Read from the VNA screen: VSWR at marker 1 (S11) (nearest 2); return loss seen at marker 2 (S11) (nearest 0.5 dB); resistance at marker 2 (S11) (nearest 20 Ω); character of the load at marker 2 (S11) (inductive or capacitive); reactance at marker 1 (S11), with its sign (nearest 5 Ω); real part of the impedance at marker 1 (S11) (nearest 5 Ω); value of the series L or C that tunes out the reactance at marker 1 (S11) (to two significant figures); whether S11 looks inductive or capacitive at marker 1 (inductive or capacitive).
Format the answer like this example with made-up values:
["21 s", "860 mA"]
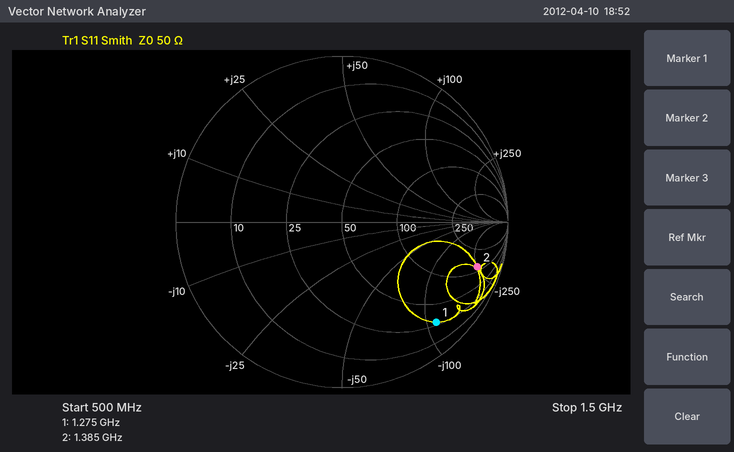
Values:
["10", "1.5 dB", "120 Ω", "capacitive", "-110 Ω", "30 Ω", "14 nH", "capacitive"]
